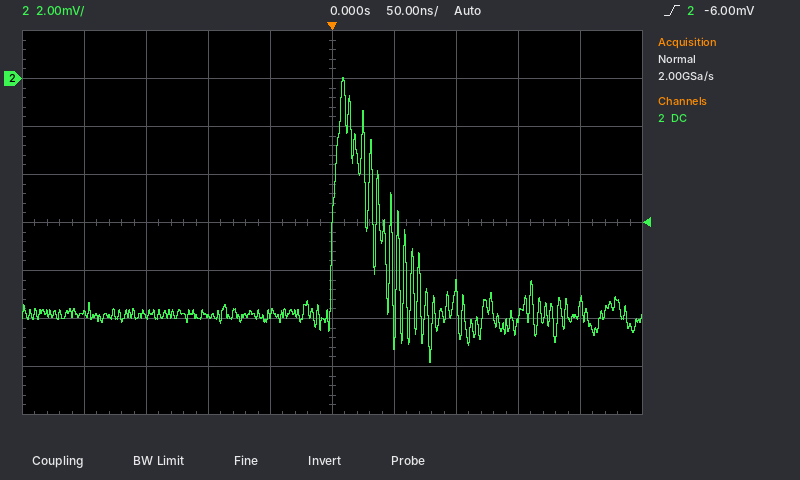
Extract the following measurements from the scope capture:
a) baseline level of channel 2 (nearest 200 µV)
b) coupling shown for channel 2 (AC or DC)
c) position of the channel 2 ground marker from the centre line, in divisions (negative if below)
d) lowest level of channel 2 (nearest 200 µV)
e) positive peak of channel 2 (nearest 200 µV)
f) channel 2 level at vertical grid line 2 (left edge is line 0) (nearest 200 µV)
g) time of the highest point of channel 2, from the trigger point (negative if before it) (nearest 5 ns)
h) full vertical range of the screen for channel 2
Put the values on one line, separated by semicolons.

-9.8 mV; DC; +3.0 div; -11.8 mV; 0.0 mV; -9.8 mV; +10 ns; 16 mV
